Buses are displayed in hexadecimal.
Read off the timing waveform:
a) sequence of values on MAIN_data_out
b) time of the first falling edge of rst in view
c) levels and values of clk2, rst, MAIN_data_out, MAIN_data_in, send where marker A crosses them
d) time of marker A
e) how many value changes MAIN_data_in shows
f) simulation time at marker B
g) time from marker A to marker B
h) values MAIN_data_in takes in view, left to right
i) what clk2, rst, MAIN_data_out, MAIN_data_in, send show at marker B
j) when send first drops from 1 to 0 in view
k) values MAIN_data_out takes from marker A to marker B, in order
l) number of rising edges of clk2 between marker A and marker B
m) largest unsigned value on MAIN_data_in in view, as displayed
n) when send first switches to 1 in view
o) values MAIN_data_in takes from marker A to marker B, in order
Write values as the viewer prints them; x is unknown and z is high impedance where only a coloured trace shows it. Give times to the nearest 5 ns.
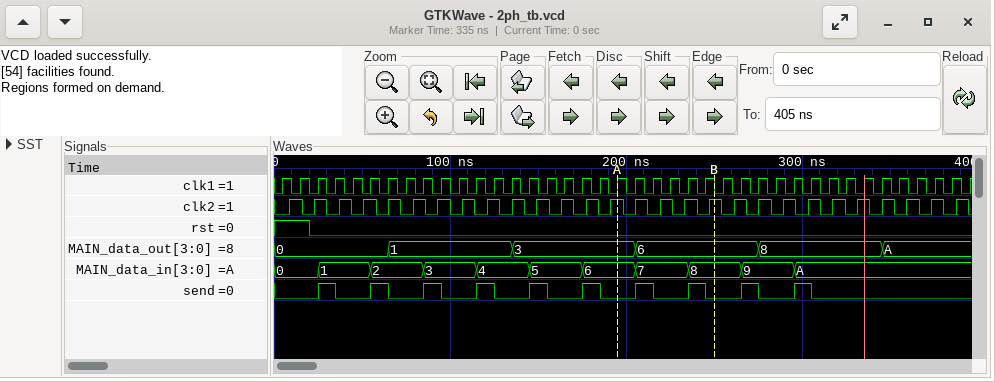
0, 1, 3, 6, 8, A
20 ns
clk2=1, rst=0, MAIN_data_out=3, MAIN_data_in=6, send=0
195 ns
10
250 ns
55 ns
0, 1, 2, 3, 4, 5, 6, 7, 8, 9, A
clk2=1, rst=0, MAIN_data_out=6, MAIN_data_in=8, send=0
35 ns
3, 6
4
A
25 ns
6, 7, 8
